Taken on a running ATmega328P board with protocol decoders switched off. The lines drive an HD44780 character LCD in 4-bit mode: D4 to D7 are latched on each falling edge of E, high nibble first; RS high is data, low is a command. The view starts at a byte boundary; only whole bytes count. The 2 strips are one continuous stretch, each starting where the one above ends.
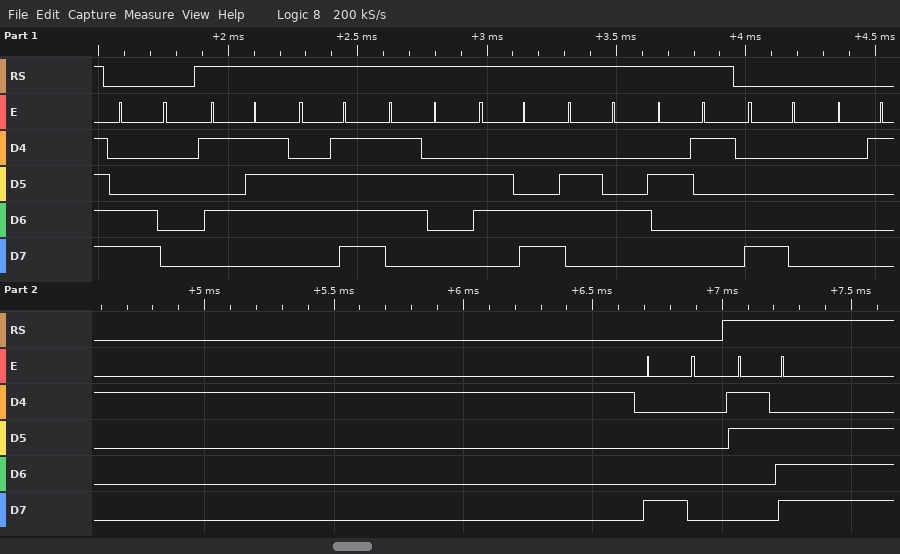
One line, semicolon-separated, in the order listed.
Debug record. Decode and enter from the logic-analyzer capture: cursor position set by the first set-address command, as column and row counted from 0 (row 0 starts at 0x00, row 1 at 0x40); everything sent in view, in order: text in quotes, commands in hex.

column 0, row 1; 0xC0 "World!" 0x80 0x01 0x80 ">"
